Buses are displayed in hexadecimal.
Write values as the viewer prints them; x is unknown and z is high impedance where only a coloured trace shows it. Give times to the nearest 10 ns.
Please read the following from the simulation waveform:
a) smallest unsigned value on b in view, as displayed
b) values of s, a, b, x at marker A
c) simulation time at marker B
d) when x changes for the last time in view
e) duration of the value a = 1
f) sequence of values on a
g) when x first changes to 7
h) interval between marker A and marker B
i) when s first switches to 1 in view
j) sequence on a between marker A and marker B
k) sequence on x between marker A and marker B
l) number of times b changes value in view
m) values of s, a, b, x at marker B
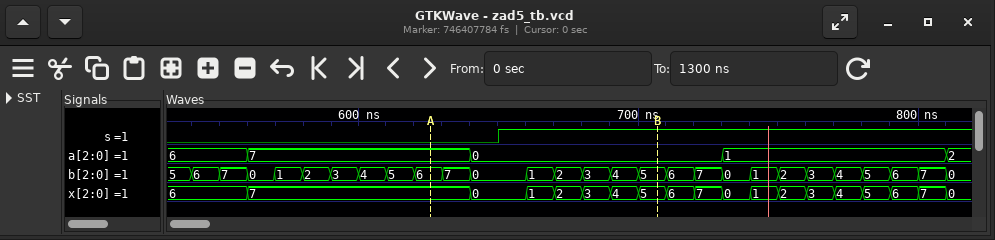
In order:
0
s=0, a=7, b=6, x=7
710 ns
810 ns
80 ns
6, 7, 0, 1, 2
560 ns
80 ns
650 ns
7, 0
7, 0, 1, 2, 3, 4, 5
27
s=1, a=0, b=5, x=5
